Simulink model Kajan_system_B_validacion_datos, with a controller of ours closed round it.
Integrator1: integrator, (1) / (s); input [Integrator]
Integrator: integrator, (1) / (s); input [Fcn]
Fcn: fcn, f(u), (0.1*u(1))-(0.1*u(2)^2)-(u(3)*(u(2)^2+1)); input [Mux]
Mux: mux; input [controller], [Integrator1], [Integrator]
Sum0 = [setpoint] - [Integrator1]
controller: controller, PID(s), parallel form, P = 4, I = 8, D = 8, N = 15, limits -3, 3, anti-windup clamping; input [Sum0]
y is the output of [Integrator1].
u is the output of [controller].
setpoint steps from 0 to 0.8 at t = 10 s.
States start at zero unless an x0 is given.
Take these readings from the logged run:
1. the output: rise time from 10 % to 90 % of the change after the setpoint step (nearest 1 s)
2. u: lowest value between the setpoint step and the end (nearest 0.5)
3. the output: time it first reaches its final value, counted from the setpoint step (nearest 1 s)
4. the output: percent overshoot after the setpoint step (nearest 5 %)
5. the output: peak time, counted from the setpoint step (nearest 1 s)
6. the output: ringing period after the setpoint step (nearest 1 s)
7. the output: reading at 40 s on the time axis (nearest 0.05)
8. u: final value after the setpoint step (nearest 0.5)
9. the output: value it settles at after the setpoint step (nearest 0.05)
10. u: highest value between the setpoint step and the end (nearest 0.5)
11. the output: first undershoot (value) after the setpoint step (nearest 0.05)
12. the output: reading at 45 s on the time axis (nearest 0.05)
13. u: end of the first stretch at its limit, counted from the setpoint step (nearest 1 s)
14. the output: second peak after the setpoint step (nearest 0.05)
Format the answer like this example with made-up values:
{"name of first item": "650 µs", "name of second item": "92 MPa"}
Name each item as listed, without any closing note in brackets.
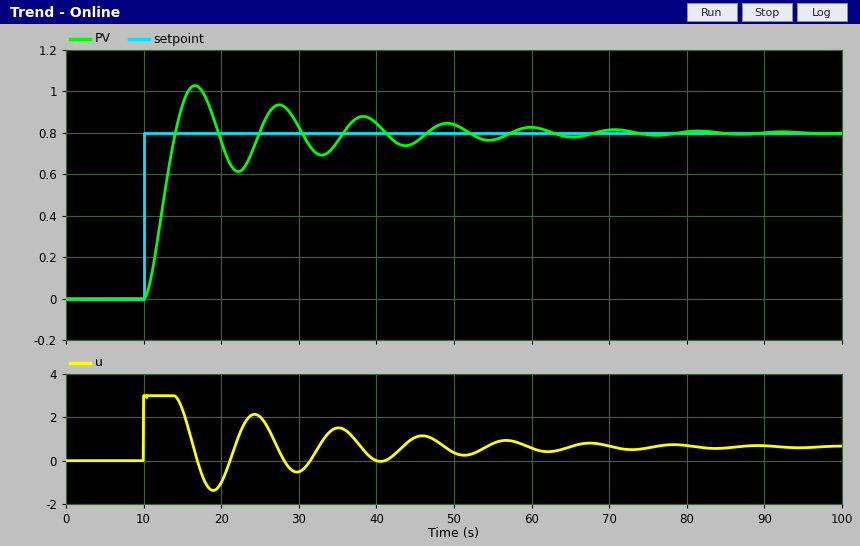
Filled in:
{"the output: rise time from 10 % to 90 % of the change after the setpoint step": "3 s", "u: lowest value between the setpoint step and the end": "-1.5", "the output: time it first reaches its final value, counted from the setpoint step": "4 s", "the output: percent overshoot after the setpoint step": "30 %", "the output: peak time, counted from the setpoint step": "7 s", "the output: ringing period after the setpoint step": "11 s", "the output: reading at 40 s on the time axis": "0.85", "u: final value after the setpoint step": "0.5", "the output: value it settles at after the setpoint step": "0.80", "u: highest value between the setpoint step and the end": "3.0", "the output: first undershoot (value) after the setpoint step": "0.60", "the output: reading at 45 s on the time axis": "0.75", "u: end of the first stretch at its limit, counted from the setpoint step": "4 s", "the output: second peak after the setpoint step": "0.95"}
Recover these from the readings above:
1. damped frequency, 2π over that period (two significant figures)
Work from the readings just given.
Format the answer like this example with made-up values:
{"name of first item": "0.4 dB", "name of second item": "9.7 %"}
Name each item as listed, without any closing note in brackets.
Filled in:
{"damped frequency, 2π over that period": "0.57 rad/s"}
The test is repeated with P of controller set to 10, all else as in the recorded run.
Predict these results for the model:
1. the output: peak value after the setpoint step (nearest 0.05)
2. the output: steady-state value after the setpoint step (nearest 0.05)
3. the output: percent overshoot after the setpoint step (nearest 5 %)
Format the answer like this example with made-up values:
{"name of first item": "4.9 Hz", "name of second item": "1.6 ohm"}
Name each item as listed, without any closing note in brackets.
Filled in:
{"the output: peak value after the setpoint step": "0.95", "the output: steady-state value after the setpoint step": "0.80", "the output: percent overshoot after the setpoint step": "20 %"}
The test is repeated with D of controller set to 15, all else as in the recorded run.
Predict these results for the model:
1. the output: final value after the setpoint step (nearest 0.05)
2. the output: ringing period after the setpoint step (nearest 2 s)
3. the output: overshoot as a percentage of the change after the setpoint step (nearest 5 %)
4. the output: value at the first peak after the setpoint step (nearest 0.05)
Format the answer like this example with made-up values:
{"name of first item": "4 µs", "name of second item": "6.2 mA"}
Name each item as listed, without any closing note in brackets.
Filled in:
{"the output: final value after the setpoint step": "0.80", "the output: ringing period after the setpoint step": "12 s", "the output: overshoot as a percentage of the change after the setpoint step": "35 %", "the output: value at the first peak after the setpoint step": "1.05"}
